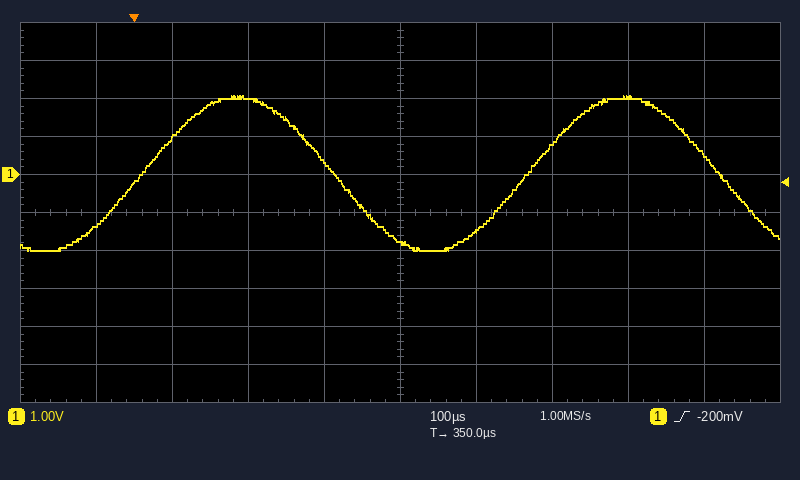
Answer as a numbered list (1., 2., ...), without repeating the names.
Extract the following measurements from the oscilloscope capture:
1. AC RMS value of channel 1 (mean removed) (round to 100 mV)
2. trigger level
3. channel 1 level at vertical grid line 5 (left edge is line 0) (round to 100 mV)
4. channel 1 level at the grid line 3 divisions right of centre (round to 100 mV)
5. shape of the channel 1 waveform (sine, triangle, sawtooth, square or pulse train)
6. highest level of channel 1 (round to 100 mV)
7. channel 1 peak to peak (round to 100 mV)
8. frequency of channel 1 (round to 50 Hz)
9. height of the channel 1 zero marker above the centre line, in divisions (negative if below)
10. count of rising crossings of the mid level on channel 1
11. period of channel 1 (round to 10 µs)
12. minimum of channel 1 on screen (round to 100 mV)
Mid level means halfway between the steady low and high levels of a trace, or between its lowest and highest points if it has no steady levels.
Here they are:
1. 1.4 V
2. -200 mV
3. -1.8 V
4. 2.0 V
5. sine
6. 2.1 V
7. 4.1 V
8. 1.95 kHz
9. +1.0 div
10. 2
11. 510 µs
12. -2.0 V
